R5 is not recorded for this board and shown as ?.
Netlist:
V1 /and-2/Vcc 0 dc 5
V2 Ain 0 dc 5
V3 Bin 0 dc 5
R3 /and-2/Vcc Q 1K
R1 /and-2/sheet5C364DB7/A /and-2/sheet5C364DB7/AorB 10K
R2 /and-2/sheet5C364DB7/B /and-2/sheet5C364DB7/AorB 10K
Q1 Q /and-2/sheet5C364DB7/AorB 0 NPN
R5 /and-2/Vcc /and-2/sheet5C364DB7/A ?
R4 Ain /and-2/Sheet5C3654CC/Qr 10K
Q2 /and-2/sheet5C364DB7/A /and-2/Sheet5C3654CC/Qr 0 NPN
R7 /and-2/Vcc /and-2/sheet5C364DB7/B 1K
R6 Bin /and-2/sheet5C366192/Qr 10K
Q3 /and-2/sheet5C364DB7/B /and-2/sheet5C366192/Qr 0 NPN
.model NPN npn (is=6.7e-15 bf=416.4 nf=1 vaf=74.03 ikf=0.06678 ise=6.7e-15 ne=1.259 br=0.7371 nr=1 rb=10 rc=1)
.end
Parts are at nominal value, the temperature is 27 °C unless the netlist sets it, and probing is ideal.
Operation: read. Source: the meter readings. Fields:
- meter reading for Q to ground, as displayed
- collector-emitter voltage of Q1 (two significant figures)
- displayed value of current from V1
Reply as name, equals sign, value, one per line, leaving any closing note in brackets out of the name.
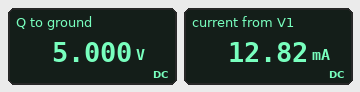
meter reading for Q to ground, as displayed = 5.000 V
collector-emitter voltage of Q1 = 5.0 V
displayed value of current from V1 = 12.82 mA
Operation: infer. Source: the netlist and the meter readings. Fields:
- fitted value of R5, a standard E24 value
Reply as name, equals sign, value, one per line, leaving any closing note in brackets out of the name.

fitted value of R5, a standard E24 value = 620 Ω
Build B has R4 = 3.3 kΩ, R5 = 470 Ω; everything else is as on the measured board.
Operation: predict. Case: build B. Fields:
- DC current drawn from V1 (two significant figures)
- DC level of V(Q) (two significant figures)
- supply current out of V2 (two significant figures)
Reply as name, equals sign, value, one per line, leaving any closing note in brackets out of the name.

DC current drawn from V1 = 15 mA
DC level of V(Q) = 5.0 V
supply current out of V2 = 1.3 mA
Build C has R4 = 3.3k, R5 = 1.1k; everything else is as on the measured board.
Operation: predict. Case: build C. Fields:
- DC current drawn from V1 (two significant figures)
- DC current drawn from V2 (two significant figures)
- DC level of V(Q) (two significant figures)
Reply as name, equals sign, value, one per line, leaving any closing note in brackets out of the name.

DC current drawn from V1 = 9.4 mA
DC current drawn from V2 = 1.3 mA
DC level of V(Q) = 5.0 V
